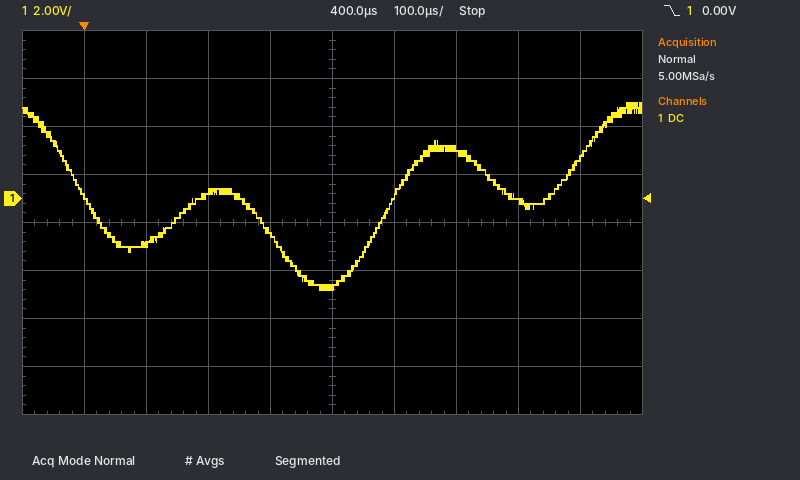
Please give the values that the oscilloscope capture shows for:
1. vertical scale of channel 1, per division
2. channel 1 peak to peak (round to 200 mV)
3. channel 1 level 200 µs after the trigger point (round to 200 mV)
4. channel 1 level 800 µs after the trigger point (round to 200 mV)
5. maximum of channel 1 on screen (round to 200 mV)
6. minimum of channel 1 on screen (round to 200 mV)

2 V
7.8 V
200 mV
1.8 V
4.0 V
-3.8 V
